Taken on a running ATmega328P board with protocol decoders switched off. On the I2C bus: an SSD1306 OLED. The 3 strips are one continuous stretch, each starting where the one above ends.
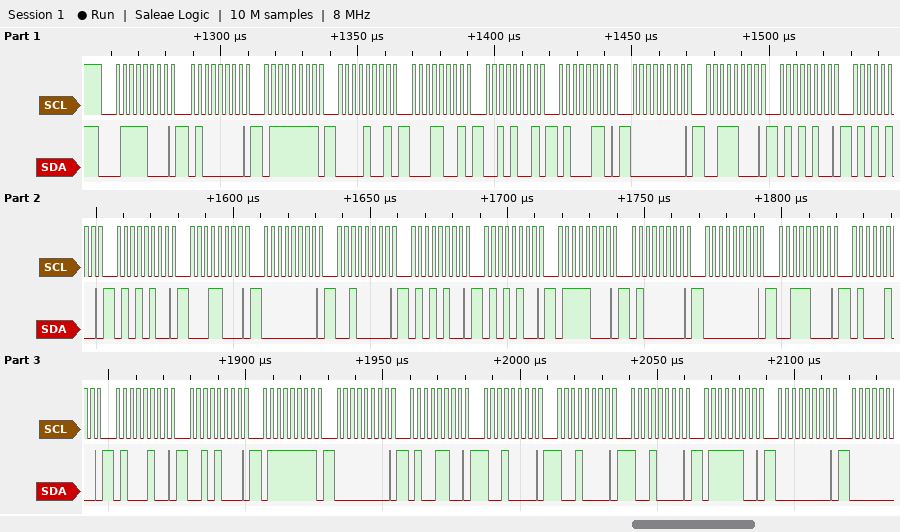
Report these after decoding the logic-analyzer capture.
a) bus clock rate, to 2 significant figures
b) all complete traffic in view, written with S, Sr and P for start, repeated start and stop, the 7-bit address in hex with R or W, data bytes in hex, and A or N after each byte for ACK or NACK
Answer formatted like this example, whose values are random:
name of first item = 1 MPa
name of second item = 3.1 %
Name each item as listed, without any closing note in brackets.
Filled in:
bus clock rate, to 2 significant figures = 400 kHz
all complete traffic in view, written with S, Sr and P for start, repeated start and stop, the 7-bit address in hex with R or W, data bytes in hex, and A or N after each byte for ACK or NACK = S 3CW A 40 A 7F A 09 A 19 A 29 A 46 A 00 A 38 A 54 A 54 A 54 A 18 A 00 A 20 A 54 A 54 A 78 A 40 A 00 A 38 A 44 A 44 A 28 A 7F A 00 A 4C A 90 A 90 A 90 A 7C A 00 A
